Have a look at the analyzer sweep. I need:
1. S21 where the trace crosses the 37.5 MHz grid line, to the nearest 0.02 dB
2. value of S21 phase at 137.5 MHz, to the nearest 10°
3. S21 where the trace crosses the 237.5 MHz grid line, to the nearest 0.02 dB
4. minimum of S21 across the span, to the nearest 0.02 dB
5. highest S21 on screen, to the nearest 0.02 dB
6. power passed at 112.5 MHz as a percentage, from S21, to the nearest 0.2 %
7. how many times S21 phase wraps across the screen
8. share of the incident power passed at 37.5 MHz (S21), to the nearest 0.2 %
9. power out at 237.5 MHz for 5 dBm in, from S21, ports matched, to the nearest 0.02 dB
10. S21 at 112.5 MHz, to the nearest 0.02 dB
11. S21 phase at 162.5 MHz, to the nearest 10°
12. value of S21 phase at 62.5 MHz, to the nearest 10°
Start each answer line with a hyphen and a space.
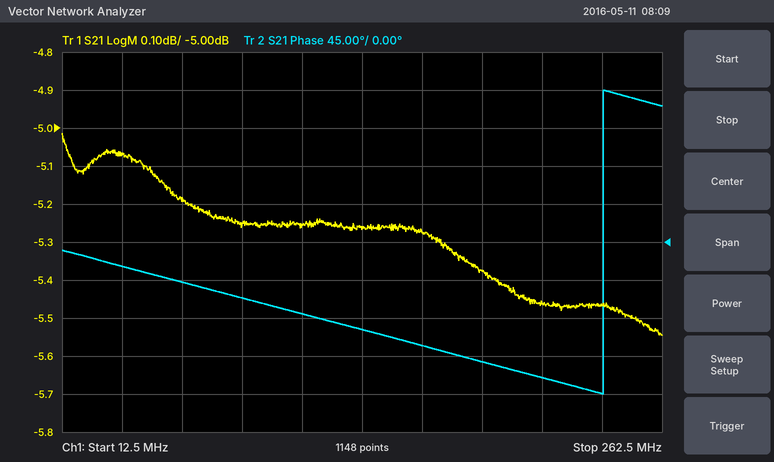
- -5.06 dB
- -100°
- -5.46 dB
- -5.54 dB
- -5.02 dB
- 29.8 %
- 1
- 31.2 %
- -0.46 dBm
- -5.26 dB
- -120°
- -50°
